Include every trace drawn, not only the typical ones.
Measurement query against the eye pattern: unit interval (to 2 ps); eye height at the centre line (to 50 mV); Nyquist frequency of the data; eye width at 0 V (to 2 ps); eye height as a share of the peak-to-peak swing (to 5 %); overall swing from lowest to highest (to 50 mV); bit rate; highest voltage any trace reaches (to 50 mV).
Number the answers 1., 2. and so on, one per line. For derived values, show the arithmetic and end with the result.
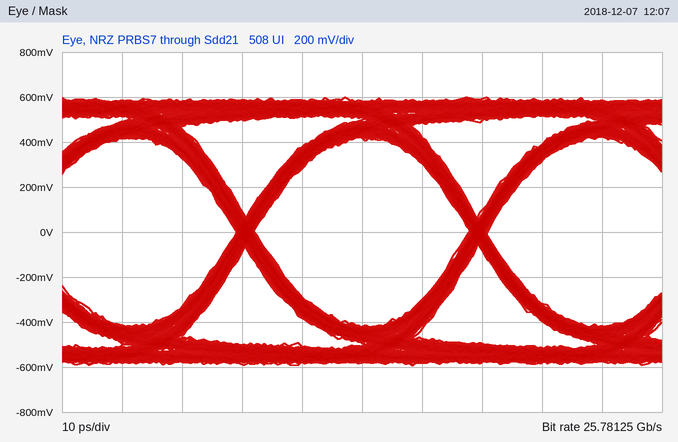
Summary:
1. 38 ps
2. 850 mV
3. 12.89062 GHz
4. 36 ps
5. 850 mV / 1.20 V ≈ 70.8 %, so 70 % to the nearest 5 %
6. 1.20 V
7. 25.78125 Gb/s
8. 600 mV
